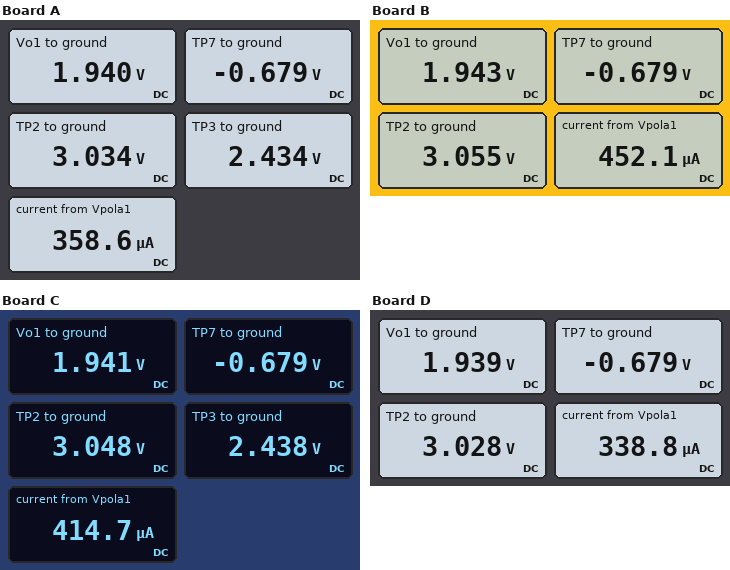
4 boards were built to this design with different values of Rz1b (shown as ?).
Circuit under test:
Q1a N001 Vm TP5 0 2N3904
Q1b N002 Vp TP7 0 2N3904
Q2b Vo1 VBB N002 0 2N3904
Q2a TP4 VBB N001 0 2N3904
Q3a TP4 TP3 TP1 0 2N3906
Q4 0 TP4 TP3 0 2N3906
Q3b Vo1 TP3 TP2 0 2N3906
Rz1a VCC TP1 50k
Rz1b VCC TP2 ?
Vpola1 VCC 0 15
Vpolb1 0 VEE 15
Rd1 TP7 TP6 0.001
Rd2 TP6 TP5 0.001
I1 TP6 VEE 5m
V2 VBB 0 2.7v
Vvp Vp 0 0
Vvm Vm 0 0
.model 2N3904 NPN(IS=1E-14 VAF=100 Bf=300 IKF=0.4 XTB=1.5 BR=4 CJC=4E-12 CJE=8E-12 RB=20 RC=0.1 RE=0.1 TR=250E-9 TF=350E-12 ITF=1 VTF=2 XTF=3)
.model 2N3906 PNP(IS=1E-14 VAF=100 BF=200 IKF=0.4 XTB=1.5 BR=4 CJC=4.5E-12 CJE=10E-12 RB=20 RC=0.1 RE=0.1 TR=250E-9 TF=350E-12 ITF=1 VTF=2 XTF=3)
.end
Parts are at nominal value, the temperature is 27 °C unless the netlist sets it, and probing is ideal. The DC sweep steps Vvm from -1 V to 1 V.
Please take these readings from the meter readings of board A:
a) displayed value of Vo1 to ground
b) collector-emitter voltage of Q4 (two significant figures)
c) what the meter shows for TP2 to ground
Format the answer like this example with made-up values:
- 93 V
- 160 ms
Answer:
- 1.940 V
- -2.4 V
- 3.034 V
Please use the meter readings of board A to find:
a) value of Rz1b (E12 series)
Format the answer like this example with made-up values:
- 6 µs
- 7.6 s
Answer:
- 100 kΩ
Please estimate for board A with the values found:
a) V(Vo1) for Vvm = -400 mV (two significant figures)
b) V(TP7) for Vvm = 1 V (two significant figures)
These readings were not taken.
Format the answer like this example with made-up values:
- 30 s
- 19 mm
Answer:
- 1.9 V
- 300 mV
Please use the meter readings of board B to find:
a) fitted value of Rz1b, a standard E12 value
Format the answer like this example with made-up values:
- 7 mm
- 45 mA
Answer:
- 56 kΩ
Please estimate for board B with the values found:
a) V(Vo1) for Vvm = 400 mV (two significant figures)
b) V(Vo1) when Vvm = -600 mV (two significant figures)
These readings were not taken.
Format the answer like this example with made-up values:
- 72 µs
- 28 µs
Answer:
- 3.1 V
- 1.9 V
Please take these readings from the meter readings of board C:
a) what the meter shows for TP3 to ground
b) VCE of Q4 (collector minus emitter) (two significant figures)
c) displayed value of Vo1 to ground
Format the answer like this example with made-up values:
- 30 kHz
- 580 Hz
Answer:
- 2.438 V
- -2.4 V
- 1.941 V
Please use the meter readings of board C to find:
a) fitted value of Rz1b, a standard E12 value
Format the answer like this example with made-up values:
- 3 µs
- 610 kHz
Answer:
- 68 kΩ
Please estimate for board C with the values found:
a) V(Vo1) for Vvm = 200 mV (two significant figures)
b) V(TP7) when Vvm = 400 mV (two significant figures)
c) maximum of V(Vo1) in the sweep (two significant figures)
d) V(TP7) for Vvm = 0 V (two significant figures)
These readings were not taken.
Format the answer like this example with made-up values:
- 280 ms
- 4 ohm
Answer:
- 3.1 V
- -300 mV
- 3.1 V
- -680 mV
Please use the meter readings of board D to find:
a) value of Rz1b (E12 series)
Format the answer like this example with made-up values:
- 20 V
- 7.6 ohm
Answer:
- 120 kΩ
